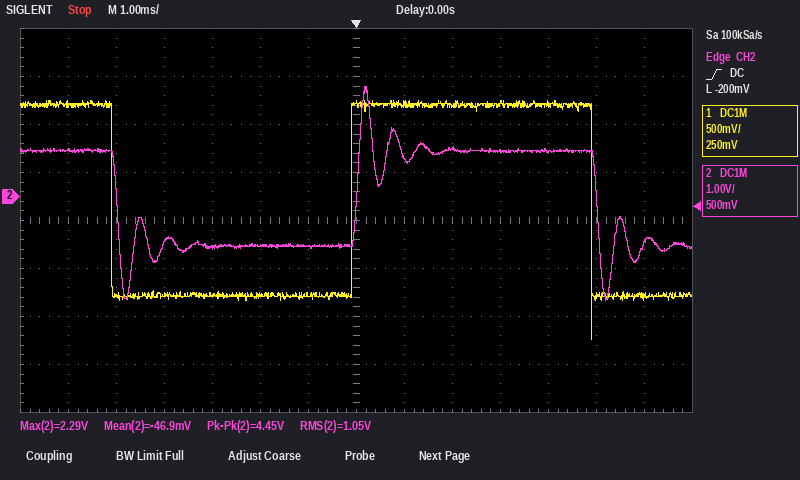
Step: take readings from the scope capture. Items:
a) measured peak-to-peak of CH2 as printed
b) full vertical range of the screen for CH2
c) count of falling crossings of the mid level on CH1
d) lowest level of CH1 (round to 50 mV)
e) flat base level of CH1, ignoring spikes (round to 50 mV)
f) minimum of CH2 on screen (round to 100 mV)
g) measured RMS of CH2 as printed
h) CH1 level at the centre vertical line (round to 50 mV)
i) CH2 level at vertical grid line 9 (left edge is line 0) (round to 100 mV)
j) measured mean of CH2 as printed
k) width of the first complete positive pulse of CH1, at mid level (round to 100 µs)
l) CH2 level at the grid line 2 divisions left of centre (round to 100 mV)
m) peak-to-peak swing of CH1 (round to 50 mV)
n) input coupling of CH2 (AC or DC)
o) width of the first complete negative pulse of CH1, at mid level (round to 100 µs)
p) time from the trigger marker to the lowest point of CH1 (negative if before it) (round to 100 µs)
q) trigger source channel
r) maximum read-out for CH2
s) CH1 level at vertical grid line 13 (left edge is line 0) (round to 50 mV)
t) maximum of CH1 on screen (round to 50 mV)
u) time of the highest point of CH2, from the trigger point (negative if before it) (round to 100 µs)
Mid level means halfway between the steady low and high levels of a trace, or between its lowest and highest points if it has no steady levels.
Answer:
4.45 V
8 V
2
-1.50 V
-1.05 V
-2.2 V
1.05 V
950 mV
1.0 V
-46.9 mV
5.0 ms
-1.0 V
2.50 V
DC
5.0 ms
+4.9 ms
CH2
2.29 V
-1.05 V
1.00 V
+200 µs
